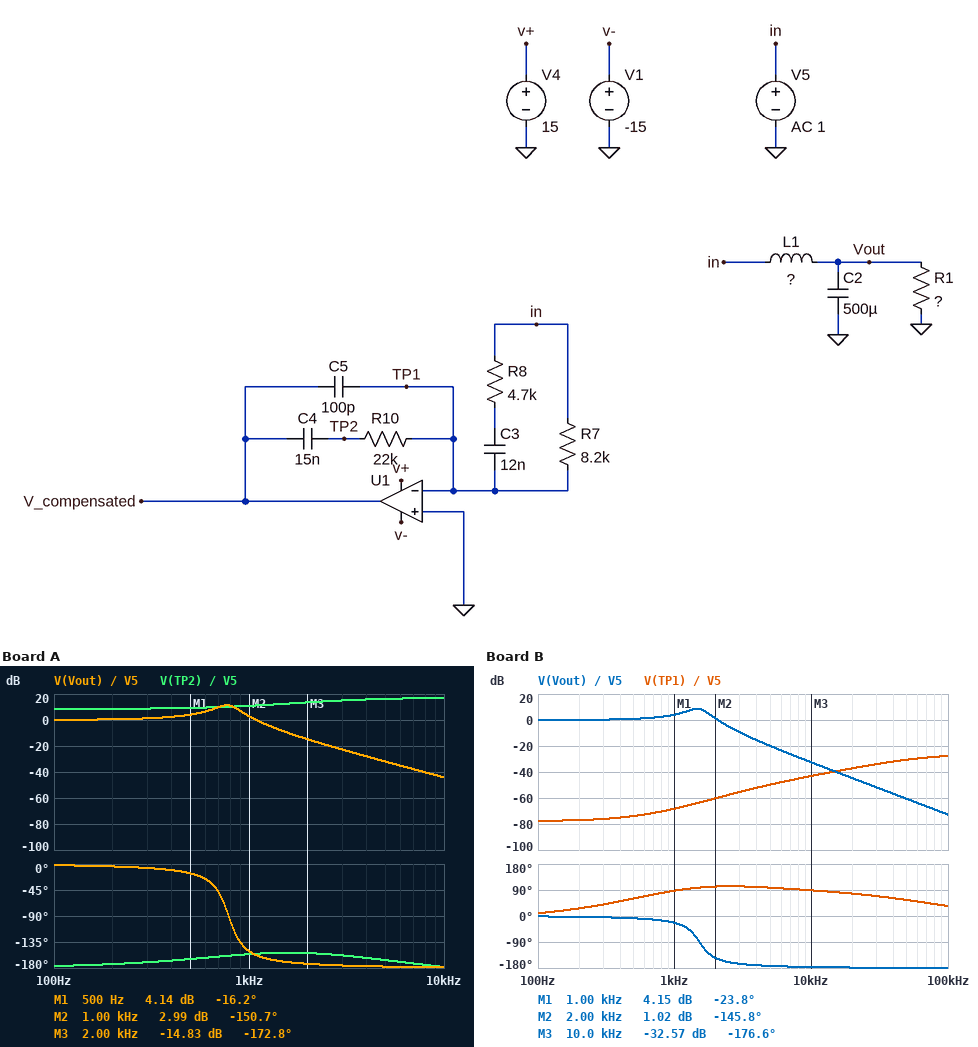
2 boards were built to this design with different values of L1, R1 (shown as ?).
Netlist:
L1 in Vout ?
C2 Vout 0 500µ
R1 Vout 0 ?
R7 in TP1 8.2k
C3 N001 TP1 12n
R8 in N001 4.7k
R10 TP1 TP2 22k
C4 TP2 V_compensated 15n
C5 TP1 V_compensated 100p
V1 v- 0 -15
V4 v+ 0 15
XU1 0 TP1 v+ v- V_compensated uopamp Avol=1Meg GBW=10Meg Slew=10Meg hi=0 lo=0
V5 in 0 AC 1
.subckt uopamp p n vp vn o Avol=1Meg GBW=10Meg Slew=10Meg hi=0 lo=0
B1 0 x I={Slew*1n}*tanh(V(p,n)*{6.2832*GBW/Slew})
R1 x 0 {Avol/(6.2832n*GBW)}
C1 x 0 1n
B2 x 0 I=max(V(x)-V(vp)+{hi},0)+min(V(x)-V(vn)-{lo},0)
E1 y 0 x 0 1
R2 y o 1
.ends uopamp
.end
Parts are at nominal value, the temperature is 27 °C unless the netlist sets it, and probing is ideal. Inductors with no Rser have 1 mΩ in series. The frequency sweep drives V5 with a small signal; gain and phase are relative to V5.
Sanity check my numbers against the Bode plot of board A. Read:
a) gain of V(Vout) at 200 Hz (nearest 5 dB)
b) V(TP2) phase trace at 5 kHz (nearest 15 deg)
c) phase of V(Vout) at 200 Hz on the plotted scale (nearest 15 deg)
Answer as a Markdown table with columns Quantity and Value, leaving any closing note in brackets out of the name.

| Quantity | Value |
|---|---|
| gain of V(Vout) at 200 Hz | 0 dB |
| V(TP2) phase trace at 5 kHz | -165 deg |
| phase of V(Vout) at 200 Hz on the plotted scale | 0 deg |
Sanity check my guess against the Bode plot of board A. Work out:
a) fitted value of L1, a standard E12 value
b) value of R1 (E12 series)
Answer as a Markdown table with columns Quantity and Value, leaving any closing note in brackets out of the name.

| Quantity | Value |
|---|---|
| fitted value of L1, a standard E12 value | 82 µH |
| value of R1 | 1.5 Ω |
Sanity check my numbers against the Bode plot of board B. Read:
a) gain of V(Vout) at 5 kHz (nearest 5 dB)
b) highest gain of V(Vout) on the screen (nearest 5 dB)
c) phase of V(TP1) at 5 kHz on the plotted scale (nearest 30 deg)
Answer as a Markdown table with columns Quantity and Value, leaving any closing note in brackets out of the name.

| Quantity | Value |
|---|---|
| gain of V(Vout) at 5 kHz | -20 dB |
| highest gain of V(Vout) on the screen | 10 dB |
| phase of V(TP1) at 5 kHz on the plotted scale | 90 deg |
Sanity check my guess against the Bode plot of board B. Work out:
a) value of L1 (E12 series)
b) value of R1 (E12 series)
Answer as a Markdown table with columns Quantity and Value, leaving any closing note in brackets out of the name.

| Quantity | Value |
|---|---|
| value of L1 | 22 µH |
| value of R1 | 0.56 Ω |
